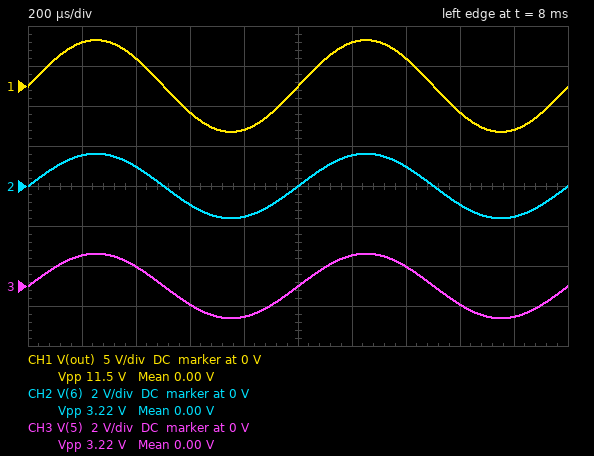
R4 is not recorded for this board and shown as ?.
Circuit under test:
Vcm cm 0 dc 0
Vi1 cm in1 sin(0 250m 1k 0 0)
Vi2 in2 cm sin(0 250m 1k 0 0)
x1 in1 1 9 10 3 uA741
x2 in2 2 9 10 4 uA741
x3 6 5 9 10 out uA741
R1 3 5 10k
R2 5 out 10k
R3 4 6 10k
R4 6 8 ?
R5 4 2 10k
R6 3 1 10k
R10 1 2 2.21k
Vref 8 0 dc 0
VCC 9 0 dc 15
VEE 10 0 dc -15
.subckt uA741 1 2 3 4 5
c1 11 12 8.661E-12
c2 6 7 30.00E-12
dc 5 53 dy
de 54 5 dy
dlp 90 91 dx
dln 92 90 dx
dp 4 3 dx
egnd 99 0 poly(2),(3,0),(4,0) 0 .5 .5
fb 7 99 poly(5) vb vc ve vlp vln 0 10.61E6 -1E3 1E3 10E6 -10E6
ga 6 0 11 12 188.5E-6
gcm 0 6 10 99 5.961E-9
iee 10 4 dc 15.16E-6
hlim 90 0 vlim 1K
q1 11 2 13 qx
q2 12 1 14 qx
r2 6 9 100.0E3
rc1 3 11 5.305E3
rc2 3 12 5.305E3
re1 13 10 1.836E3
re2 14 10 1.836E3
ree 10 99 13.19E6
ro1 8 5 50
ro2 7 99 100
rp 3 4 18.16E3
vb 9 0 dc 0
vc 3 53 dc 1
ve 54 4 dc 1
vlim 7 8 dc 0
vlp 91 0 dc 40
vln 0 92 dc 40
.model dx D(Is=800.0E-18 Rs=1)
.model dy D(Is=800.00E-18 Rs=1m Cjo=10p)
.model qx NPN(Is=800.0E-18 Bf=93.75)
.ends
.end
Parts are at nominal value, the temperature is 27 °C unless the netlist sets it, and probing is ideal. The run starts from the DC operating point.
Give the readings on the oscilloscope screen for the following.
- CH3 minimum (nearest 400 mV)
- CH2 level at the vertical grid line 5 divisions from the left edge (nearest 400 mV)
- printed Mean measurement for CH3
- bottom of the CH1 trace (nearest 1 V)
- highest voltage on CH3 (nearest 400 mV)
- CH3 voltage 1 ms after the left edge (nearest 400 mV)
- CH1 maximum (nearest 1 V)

-1.6 V
0 V
0.00 V
-6 V
1.6 V
0 V
6 V
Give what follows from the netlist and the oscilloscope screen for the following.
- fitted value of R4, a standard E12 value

18 kΩ
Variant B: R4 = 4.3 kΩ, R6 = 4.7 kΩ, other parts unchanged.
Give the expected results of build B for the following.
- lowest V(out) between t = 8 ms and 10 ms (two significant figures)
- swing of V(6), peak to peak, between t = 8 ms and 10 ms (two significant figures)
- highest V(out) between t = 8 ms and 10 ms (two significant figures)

-2.8 V
1.5 V
2.8 V
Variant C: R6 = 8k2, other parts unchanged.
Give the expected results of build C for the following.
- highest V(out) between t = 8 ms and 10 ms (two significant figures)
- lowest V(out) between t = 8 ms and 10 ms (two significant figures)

5.3 V
-5.3 V
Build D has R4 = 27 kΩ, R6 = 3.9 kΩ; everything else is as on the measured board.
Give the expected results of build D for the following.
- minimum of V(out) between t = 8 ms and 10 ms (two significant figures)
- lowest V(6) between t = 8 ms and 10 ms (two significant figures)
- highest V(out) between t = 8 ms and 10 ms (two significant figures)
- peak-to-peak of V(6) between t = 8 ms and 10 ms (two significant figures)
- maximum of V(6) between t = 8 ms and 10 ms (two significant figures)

-4.8 V
-1.8 V
4.8 V
3.7 V
1.8 V
